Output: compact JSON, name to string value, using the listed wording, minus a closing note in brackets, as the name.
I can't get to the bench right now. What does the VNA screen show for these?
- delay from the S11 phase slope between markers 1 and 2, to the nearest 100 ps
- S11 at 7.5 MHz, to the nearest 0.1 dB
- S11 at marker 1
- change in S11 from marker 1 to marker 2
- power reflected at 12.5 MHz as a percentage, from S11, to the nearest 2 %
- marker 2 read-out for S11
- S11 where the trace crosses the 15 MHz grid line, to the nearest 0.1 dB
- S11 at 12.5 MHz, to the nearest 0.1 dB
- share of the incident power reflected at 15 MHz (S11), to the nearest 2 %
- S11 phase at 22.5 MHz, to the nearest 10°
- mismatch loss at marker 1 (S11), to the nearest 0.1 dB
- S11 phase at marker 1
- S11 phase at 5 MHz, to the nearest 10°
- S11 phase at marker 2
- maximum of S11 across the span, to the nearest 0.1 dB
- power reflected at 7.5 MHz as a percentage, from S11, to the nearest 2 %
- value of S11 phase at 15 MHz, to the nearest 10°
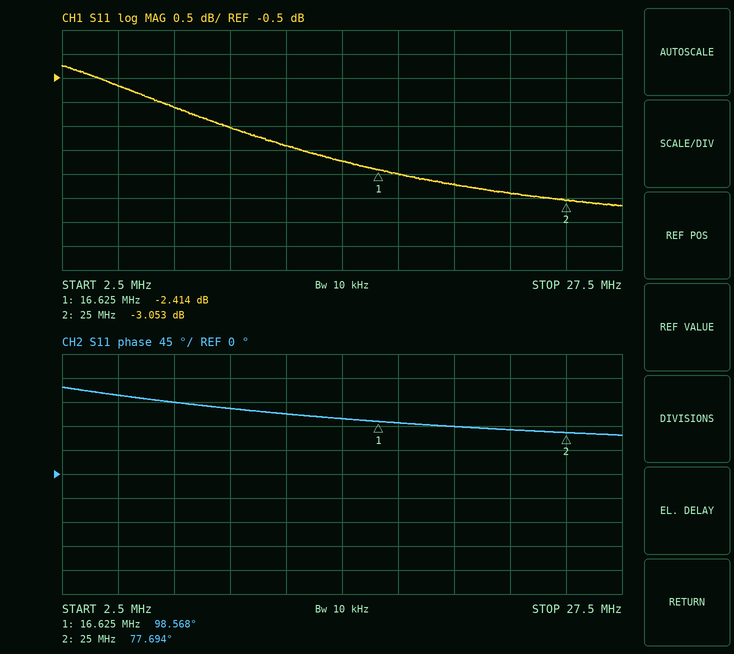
{"delay from the S11 phase slope between markers 1 and 2, to the nearest 100 ps": "6.9 ns", "S11 at 7.5 MHz, to the nearest 0.1 dB": "-1.1 dB", "S11 at marker 1": "-2.414 dB", "change in S11 from marker 1 to marker 2": "-0.639 dB", "power reflected at 12.5 MHz as a percentage, from S11, to the nearest 2 %": "64 %", "marker 2 read-out for S11": "-3.053 dB", "S11 where the trace crosses the 15 MHz grid line, to the nearest 0.1 dB": "-2.2 dB", "S11 at 12.5 MHz, to the nearest 0.1 dB": "-1.9 dB", "share of the incident power reflected at 15 MHz (S11), to the nearest 2 %": "60 %", "S11 phase at 22.5 MHz, to the nearest 10°": "80°", "mismatch loss at marker 1 (S11), to the nearest 0.1 dB": "3.7 dB", "S11 phase at marker 1": "98.568°", "S11 phase at 5 MHz, to the nearest 10°": "150°", "S11 phase at marker 2": "77.694°", "maximum of S11 across the span, to the nearest 0.1 dB": "-0.2 dB", "power reflected at 7.5 MHz as a percentage, from S11, to the nearest 2 %": "78 %", "value of S11 phase at 15 MHz, to the nearest 10°": "100°"}
